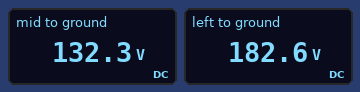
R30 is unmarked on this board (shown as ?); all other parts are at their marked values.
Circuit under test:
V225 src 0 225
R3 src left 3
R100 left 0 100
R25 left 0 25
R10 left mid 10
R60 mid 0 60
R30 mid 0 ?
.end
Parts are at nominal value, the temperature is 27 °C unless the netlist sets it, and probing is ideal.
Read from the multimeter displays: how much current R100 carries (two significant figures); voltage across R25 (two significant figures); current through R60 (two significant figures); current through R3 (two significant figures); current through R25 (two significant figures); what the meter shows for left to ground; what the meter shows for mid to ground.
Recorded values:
1.8 A
180 V
2.2 A
14 A
7.3 A
182.6 V
132.3 V
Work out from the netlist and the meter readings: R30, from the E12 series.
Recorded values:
47 Ω
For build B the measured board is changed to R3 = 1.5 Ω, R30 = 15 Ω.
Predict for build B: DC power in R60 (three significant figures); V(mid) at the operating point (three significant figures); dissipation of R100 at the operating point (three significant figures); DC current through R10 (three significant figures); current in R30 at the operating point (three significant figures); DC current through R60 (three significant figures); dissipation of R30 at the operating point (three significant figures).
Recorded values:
192 W
107 V
387 W
8.95 A
7.16 A
1.79 A
768 W
